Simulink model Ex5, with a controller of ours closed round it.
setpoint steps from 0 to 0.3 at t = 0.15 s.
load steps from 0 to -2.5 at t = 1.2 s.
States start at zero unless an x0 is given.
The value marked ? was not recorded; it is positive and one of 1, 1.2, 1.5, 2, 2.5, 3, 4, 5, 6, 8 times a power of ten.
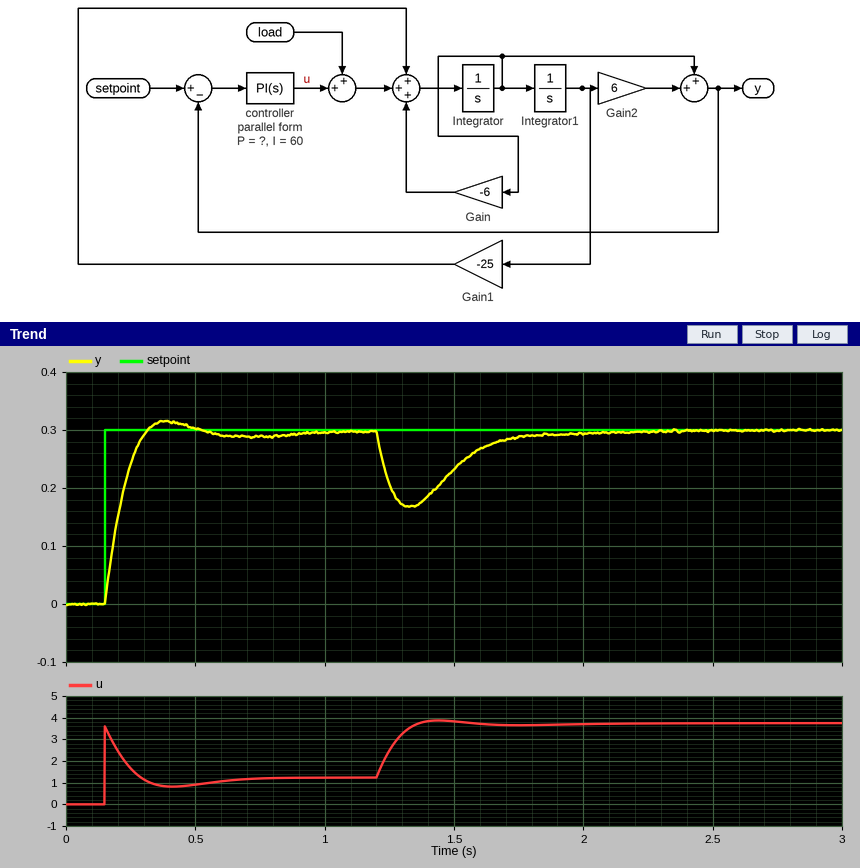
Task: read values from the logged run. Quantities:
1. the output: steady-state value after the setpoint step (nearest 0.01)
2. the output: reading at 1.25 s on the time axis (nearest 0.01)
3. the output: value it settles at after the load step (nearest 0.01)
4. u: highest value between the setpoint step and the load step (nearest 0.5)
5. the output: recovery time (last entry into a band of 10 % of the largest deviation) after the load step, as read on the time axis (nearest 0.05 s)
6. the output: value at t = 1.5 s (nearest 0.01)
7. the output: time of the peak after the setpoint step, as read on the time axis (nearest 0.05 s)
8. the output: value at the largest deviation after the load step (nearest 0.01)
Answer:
0.30
0.21
0.30
3.5
1.75 s
0.23
0.40 s
0.17
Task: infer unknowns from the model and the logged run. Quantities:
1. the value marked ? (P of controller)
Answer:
12
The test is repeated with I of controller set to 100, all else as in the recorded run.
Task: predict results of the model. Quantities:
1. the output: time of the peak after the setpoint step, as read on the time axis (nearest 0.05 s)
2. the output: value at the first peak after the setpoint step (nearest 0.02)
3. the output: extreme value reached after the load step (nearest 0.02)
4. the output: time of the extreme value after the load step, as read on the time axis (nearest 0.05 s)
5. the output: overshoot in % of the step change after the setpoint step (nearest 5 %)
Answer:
0.35 s
0.34
0.18
1.30 s
15 %
